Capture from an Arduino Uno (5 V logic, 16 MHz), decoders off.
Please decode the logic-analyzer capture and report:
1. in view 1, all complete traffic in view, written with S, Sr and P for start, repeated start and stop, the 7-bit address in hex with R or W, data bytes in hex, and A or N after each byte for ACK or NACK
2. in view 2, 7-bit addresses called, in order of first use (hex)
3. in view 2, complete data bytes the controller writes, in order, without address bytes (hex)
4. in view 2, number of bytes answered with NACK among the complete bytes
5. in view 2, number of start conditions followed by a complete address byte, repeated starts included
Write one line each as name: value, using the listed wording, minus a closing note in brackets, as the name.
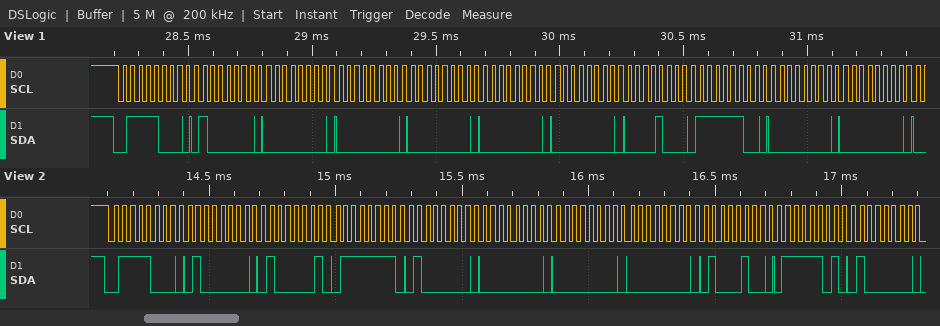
in view 1, all complete traffic in view, written with S, Sr and P for start, repeated start and stop, the 7-bit address in hex with R or W, data bytes in hex, and A or N after each byte for ACK or NACK: S 3CW A 40 A 00 A 00 A 00 A 00 A 00 A 08 A FC A 00 A 00 A
in view 2, 7-bit addresses called, in order of first use: 0x3C
in view 2, complete data bytes the controller writes, in order, without address bytes: 40 41 7F 40 00 00 00 44 7D 40
in view 2, number of bytes answered with NACK among the complete bytes: 0
in view 2, number of start conditions followed by a complete address byte, repeated starts included: 1
